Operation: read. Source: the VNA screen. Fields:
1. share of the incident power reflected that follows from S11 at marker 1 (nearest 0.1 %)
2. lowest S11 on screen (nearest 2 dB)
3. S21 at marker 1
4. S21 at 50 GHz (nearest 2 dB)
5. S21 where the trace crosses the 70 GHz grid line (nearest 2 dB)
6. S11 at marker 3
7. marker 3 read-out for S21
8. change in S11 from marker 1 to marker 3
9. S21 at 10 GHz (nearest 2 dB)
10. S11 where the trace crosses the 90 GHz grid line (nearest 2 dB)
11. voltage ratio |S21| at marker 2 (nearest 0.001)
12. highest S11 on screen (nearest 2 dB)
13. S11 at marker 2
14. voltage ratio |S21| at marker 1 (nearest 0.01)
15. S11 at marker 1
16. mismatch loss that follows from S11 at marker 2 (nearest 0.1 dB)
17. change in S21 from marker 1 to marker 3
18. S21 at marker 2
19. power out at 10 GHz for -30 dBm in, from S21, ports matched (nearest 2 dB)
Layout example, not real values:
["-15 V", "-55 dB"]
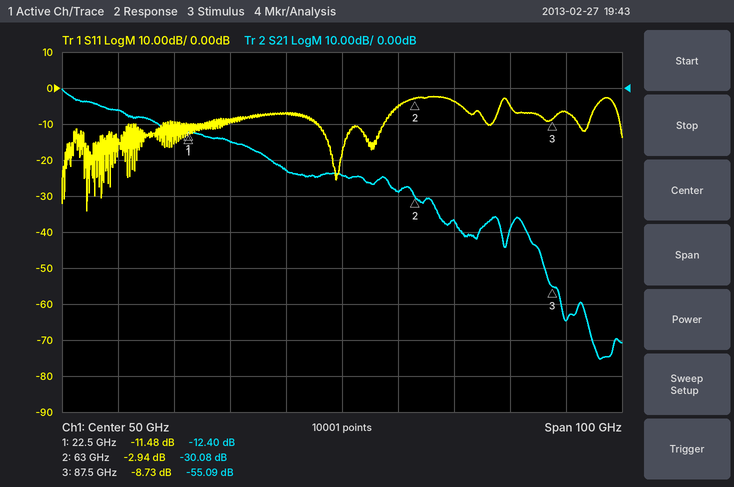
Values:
["7.1 %", "-34 dB", "-12.40 dB", "-24 dB", "-36 dB", "-8.73 dB", "-55.09 dB", "2.75 dB", "-6 dB", "-6 dB", "0.031", "-2 dB", "-2.94 dB", "0.24", "-11.48 dB", "3.1 dB", "-42.69 dB", "-30.08 dB", "-36 dBm"]
